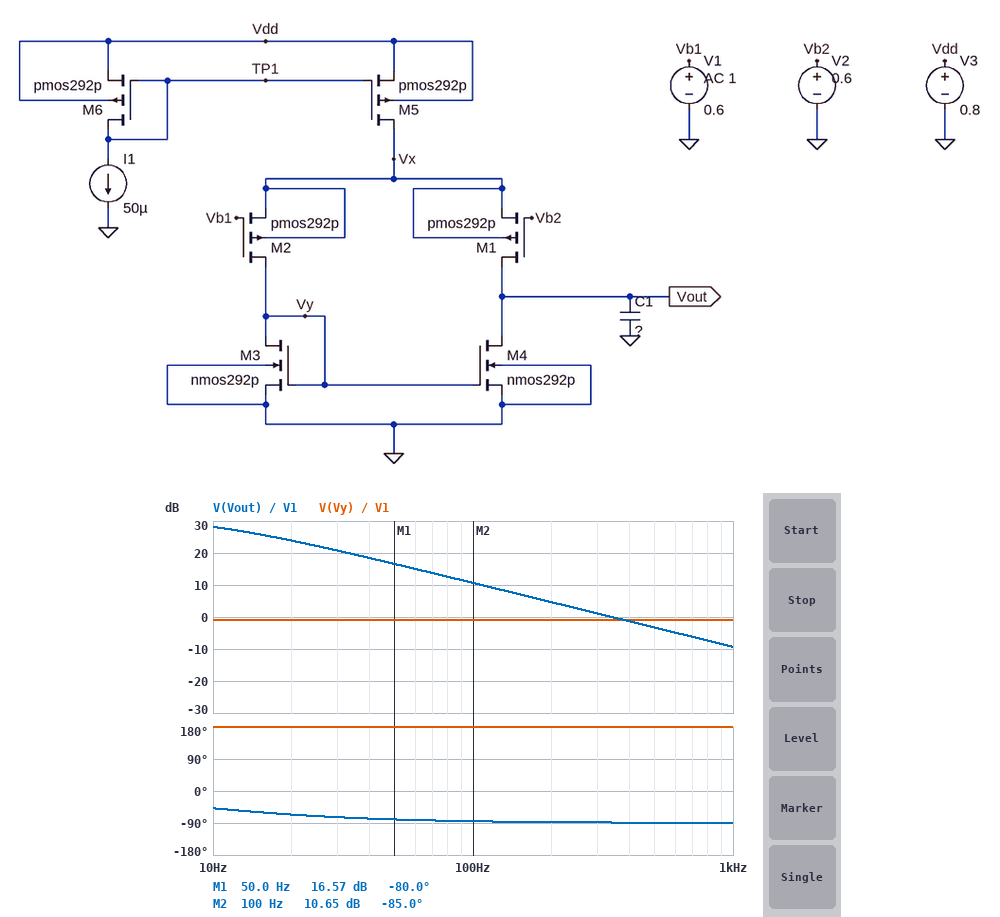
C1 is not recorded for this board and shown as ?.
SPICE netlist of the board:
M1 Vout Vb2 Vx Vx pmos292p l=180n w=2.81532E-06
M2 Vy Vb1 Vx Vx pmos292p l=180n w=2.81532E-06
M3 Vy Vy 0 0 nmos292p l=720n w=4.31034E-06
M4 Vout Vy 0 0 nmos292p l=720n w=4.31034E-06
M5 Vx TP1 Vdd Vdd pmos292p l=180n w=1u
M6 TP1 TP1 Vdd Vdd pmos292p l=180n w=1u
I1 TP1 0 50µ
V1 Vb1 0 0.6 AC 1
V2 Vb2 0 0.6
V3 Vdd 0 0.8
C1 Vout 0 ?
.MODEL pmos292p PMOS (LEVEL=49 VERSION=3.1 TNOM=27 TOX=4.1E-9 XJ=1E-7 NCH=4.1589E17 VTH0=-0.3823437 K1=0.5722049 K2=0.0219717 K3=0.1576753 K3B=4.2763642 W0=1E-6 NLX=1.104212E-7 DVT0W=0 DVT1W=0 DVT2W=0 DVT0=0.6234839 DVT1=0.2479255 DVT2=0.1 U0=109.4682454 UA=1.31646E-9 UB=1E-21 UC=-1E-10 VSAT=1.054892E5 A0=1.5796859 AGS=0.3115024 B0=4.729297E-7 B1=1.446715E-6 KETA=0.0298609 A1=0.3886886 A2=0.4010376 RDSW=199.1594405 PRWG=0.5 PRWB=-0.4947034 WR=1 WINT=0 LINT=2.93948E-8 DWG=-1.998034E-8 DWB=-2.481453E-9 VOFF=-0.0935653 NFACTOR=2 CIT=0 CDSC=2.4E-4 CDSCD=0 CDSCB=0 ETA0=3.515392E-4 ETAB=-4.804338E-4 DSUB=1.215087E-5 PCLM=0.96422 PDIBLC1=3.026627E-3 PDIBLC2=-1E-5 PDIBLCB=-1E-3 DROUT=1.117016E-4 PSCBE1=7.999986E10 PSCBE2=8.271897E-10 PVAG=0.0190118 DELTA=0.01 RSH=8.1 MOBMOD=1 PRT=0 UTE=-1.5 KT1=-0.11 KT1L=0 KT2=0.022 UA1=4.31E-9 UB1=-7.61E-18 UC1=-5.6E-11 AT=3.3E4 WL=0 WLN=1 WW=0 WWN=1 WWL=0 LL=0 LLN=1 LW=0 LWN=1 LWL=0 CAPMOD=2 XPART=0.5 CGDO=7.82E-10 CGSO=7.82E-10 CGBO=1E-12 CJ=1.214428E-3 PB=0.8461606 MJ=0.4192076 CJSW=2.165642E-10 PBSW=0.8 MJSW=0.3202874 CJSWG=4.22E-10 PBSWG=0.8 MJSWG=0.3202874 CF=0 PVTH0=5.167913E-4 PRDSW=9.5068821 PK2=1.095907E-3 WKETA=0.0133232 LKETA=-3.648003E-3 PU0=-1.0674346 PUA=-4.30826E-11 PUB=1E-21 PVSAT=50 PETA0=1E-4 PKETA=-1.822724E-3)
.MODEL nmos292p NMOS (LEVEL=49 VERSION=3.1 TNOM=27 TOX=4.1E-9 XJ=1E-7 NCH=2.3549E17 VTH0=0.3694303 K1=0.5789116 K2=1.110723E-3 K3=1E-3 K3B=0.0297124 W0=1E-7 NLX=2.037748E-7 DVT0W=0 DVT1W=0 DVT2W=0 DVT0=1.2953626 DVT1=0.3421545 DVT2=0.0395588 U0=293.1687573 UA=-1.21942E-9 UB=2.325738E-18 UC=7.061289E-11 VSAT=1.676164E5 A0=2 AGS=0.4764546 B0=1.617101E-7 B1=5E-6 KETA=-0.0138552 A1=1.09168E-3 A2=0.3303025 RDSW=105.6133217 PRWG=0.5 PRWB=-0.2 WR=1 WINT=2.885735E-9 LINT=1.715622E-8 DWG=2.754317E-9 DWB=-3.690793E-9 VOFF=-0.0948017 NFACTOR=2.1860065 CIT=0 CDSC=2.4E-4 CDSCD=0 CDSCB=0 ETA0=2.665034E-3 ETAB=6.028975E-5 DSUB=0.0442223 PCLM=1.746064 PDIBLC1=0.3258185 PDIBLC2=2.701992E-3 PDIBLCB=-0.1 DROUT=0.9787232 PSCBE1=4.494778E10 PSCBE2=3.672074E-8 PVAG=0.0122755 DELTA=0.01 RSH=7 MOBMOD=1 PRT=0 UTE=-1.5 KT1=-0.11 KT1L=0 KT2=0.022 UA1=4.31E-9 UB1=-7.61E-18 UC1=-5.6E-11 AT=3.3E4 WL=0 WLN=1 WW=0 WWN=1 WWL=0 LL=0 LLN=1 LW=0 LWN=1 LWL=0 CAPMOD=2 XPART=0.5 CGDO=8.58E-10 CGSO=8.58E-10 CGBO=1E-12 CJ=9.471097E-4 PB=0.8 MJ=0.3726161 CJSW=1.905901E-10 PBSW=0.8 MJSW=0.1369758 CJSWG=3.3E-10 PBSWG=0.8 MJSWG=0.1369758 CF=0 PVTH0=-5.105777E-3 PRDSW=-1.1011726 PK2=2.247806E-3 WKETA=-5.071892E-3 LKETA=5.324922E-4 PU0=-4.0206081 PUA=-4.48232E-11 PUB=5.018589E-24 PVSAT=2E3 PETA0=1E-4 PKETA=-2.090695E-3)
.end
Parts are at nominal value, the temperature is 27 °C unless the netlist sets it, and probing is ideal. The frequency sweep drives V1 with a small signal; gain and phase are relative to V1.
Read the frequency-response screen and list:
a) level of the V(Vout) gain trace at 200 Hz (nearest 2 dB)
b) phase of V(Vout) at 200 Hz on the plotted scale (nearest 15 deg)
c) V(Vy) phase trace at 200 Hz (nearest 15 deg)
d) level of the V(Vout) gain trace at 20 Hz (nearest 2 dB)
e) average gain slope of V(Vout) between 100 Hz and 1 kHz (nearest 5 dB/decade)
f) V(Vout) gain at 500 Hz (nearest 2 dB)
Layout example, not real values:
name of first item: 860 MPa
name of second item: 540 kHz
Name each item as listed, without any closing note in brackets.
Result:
level of the V(Vout) gain trace at 200 Hz: 4 dB
phase of V(Vout) at 200 Hz on the plotted scale: -90 deg
V(Vy) phase trace at 200 Hz: 180 deg
level of the V(Vout) gain trace at 20 Hz: 24 dB
average gain slope of V(Vout) between 100 Hz and 1 kHz: -20 dB/decade
V(Vout) gain at 500 Hz: -4 dB
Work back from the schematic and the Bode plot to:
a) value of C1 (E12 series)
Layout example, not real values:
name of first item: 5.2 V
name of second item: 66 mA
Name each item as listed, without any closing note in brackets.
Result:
value of C1: 22 pF
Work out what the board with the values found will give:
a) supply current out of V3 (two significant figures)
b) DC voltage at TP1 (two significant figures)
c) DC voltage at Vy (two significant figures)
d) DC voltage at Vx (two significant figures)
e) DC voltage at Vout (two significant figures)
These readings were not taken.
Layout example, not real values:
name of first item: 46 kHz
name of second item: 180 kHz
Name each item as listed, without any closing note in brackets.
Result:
supply current out of V3: 50 µA
DC voltage at TP1: -150 mV
DC voltage at Vy: 190 mV
DC voltage at Vx: 800 mV
DC voltage at Vout: 190 mV
